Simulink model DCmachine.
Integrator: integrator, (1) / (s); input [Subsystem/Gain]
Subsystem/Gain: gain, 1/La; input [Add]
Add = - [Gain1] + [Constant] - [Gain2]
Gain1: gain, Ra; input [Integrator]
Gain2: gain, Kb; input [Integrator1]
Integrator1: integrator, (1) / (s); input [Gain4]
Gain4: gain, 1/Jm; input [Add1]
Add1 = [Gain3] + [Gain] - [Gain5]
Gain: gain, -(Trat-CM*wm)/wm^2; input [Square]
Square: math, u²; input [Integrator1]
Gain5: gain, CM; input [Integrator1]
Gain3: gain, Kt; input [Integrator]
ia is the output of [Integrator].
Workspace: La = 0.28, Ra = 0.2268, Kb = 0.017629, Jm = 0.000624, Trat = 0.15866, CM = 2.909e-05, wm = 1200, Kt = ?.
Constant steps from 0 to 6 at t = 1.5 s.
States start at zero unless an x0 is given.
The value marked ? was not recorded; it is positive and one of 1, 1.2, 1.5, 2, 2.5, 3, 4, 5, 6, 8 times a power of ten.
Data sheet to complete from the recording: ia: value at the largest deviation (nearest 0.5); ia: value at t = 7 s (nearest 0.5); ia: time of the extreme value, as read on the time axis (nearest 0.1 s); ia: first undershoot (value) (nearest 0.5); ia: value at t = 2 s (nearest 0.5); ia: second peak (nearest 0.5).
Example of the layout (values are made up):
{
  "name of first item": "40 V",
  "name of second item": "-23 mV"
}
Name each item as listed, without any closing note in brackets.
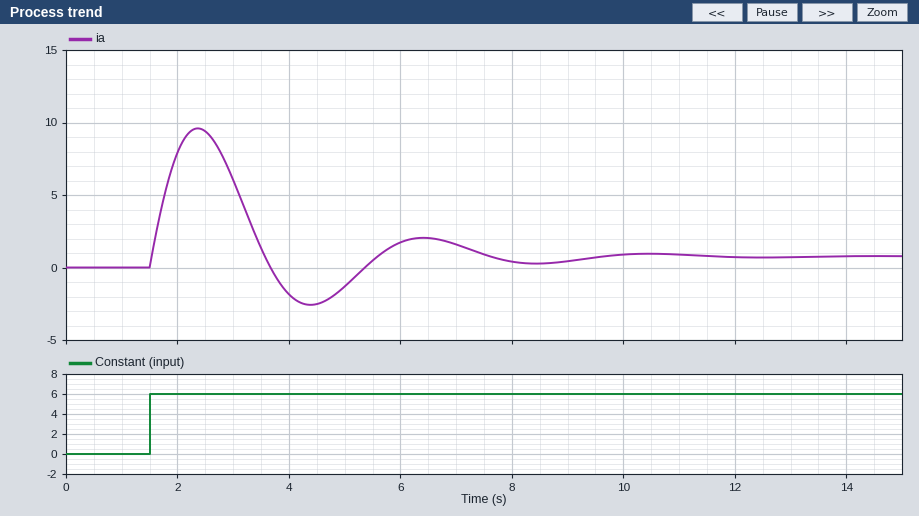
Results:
{
  "ia: value at the largest deviation": "9.5",
  "ia: value at t = 7 s": "1.5",
  "ia: time of the extreme value, as read on the time axis": "2.4 s",
  "ia: first undershoot (value)": "-2.5",
  "ia: value at t = 2 s": "8.0",
  "ia: second peak": "2.0"
}
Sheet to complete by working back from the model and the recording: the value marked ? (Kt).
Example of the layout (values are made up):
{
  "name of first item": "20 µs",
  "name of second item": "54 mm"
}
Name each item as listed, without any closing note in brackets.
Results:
{
  "the value marked ?": "0.025"
}
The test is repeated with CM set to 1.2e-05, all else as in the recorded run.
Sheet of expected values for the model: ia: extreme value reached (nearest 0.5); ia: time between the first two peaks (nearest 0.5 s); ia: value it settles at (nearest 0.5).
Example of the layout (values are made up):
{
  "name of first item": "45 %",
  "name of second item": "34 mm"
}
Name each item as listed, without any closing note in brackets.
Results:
{
  "ia: extreme value reached": "9.5",
  "ia: time between the first two peaks": "4.0 s",
  "ia: value it settles at": "0.5"
}
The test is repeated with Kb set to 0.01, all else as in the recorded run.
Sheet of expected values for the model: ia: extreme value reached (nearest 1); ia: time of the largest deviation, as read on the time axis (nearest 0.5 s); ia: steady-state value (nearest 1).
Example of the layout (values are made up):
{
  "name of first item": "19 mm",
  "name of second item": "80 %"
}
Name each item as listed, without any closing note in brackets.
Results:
{
  "ia: extreme value reached": "12",
  "ia: time of the largest deviation, as read on the time axis": "2.5 s",
  "ia: steady-state value": "2"
}
